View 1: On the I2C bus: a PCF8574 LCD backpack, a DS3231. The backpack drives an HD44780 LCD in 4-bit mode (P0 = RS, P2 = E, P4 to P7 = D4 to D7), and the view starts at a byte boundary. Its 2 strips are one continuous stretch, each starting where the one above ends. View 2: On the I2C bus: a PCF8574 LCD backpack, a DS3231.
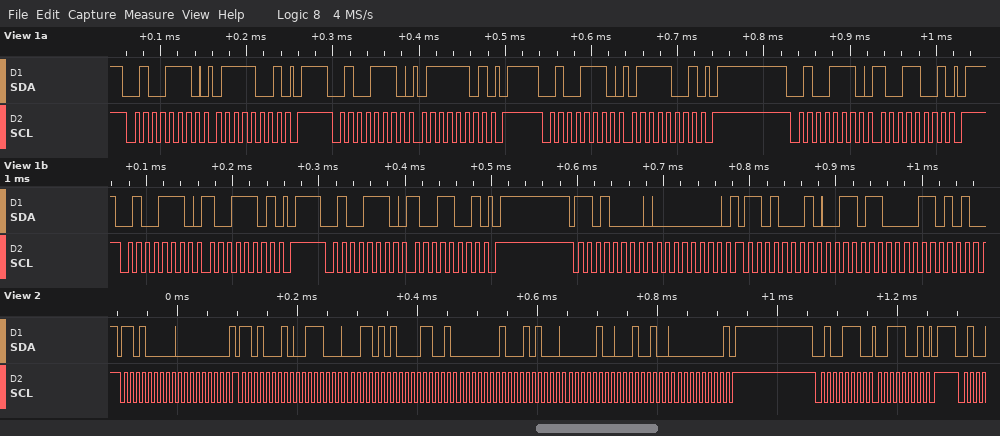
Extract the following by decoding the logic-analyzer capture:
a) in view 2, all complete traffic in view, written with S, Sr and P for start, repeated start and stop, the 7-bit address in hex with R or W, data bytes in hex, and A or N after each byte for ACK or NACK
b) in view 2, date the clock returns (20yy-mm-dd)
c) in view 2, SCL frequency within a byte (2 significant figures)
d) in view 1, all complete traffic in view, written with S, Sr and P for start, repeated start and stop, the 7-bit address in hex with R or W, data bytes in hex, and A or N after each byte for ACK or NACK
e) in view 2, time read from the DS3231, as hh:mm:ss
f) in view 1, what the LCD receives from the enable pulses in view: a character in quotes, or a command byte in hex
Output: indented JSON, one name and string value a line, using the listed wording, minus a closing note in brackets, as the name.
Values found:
{
  "in view 2, all complete traffic in view, written with S, Sr and P for start, repeated start and stop, the 7-bit address in hex with R or W, data bytes in hex, and A or N after each byte for ACK or NACK": "S 68W A 00 A Sr 68R A 38 A 35 A 19 A 01 A 28 A 04 A 24 A 00 N P S 27W A 39 A P",
  "in view 2, date the clock returns": "2024-04-28",
  "in view 2, SCL frequency within a byte": "100 kHz",
  "in view 1, all complete traffic in view, written with S, Sr and P for start, repeated start and stop, the 7-bit address in hex with R or W, data bytes in hex, and A or N after each byte for ACK or NACK": "S 27W A 79 A P S 27W A 7D A P S 27W A 79 A P S 27W A 99 A P S 27W A 9D A P S 27W A 99 A P S 68W A 00 A Sr 68R A 36 A 35 A",
  "in view 2, time read from the DS3231, as hh:mm:ss": "19:35:38",
  "in view 1, what the LCD receives from the enable pulses in view: a character in quotes, or a command byte in hex": "'y'"
}
